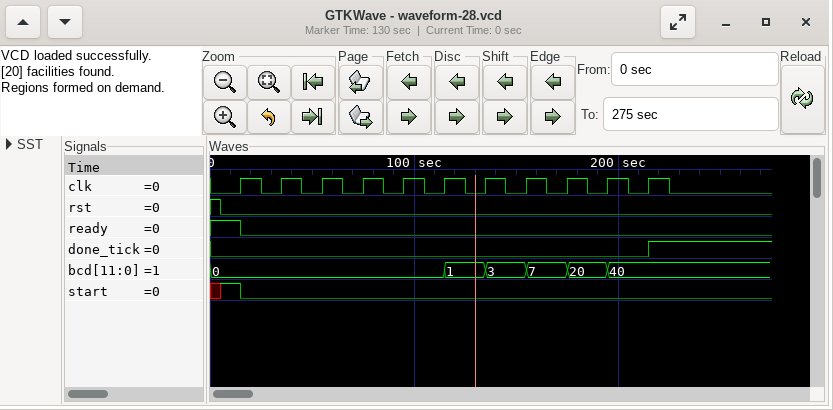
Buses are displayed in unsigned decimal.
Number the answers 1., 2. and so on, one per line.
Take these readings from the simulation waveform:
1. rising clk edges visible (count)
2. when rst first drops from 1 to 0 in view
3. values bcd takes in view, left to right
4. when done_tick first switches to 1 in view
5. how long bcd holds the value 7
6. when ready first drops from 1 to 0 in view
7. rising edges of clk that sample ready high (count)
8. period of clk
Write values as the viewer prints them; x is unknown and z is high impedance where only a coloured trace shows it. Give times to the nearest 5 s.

1. 11
2. 5 s
3. 0, 1, 3, 7, 20, 40
4. 215 s
5. 20 s
6. 15 s
7. 1
8. 20 s
